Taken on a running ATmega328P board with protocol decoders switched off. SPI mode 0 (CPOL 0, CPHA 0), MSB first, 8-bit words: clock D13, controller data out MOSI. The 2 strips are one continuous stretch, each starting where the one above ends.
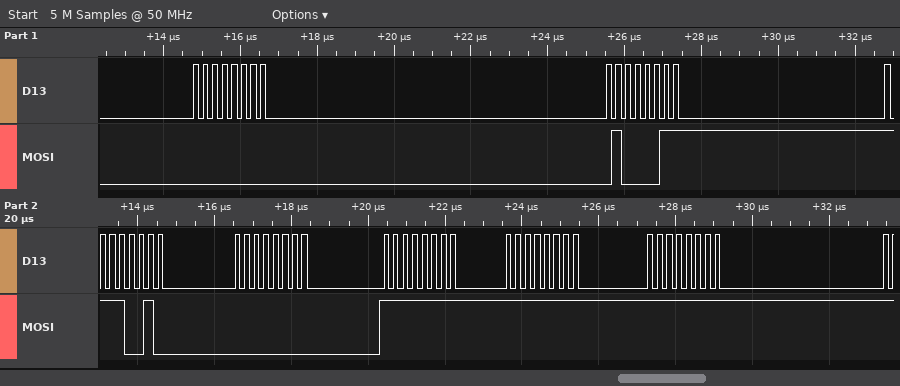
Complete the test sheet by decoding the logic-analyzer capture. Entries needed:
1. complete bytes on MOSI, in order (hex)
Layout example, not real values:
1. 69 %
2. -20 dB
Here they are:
1. 00 43 F2 00 FF FF FF
